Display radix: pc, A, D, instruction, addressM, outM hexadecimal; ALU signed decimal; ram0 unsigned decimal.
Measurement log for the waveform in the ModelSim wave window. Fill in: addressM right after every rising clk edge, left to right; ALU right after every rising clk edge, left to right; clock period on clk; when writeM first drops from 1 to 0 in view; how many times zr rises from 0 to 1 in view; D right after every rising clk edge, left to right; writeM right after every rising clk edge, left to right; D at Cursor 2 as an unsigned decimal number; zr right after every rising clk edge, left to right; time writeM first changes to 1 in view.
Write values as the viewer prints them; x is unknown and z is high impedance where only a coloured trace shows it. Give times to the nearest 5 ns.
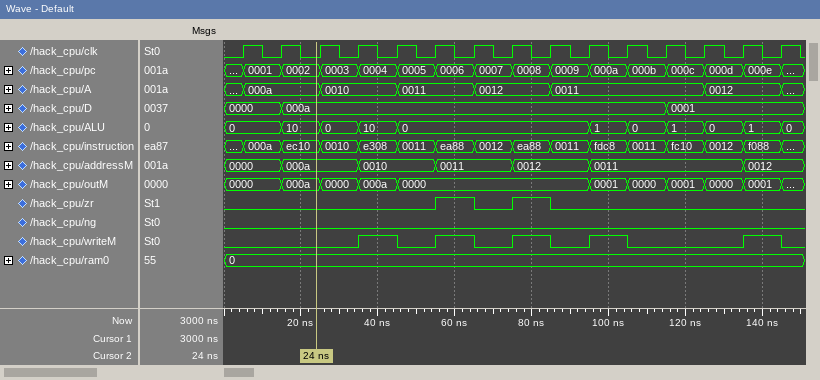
0000, 000a, 000a, 0010, 0010, 0011, 0011, 0012, 0012, 0011, 0011, 0011, 0011, 0012, 0012
0, 10, 0, 10, 0, 0, 0, 0, 0, 1, 0, 1, 0, 1, 0
10 ns
45 ns
2
0000, 000a, 000a, 000a, 000a, 000a, 000a, 000a, 000a, 000a, 000a, 0001, 0001, 0001, 0001
0 0 0 1 0 1 0 1 0 1 0 0 0 1 0
10
0 0 0 0 0 1 0 1 0 0 0 0 0 0 0
35 ns
